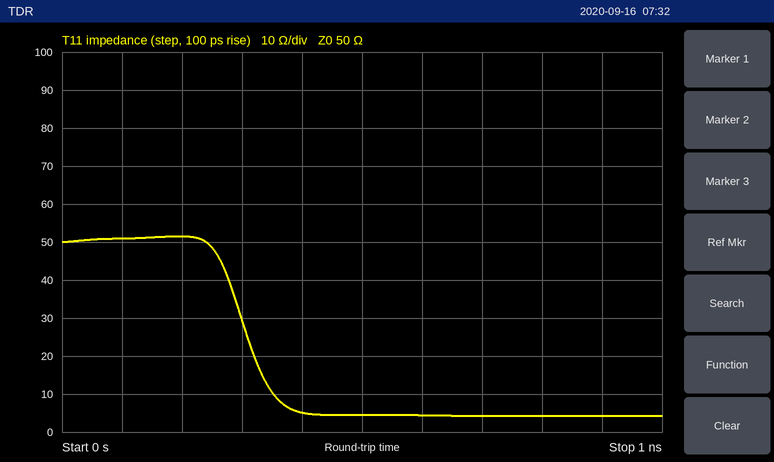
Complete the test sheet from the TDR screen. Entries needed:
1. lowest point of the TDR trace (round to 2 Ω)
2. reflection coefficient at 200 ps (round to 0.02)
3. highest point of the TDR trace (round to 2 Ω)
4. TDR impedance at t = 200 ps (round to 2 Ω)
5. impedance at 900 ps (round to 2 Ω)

4 Ω
+0.02
52 Ω
52 Ω
4 Ω
